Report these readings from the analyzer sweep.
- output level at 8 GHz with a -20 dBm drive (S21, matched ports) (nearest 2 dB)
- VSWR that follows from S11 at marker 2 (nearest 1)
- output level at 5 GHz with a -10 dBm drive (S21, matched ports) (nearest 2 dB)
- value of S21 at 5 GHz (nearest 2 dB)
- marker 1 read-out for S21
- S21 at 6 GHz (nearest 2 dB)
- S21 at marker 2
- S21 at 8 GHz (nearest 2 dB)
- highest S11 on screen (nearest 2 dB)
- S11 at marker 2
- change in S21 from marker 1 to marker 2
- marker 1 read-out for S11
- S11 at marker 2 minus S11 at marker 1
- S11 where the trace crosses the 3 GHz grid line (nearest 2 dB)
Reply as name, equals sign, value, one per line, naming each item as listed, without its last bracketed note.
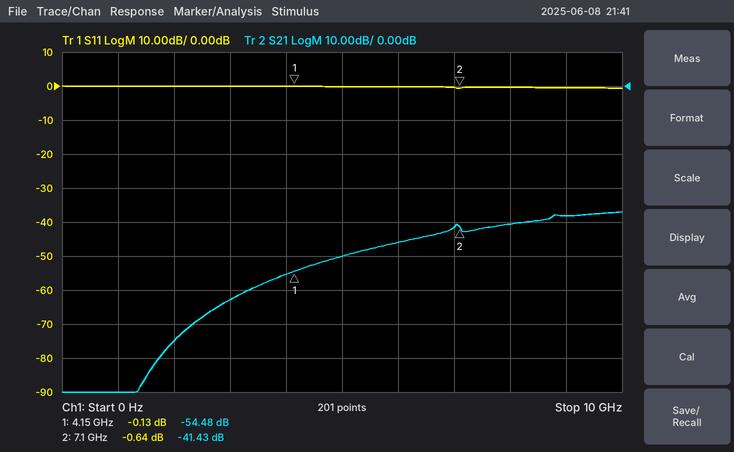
output level at 8 GHz with a -20 dBm drive (S21, matched ports) = -60 dBm
VSWR that follows from S11 at marker 2 = 27
output level at 5 GHz with a -10 dBm drive (S21, matched ports) = -60 dBm
value of S21 at 5 GHz = -50 dB
marker 1 read-out for S21 = -54.48 dB
S21 at 6 GHz = -46 dB
S21 at marker 2 = -41.43 dB
S21 at 8 GHz = -40 dB
highest S11 on screen = 0 dB
S11 at marker 2 = -0.64 dB
change in S21 from marker 1 to marker 2 = 13.05 dB
marker 1 read-out for S11 = -0.13 dB
S11 at marker 2 minus S11 at marker 1 = -0.51 dB
S11 where the trace crosses the 3 GHz grid line = 0 dB
